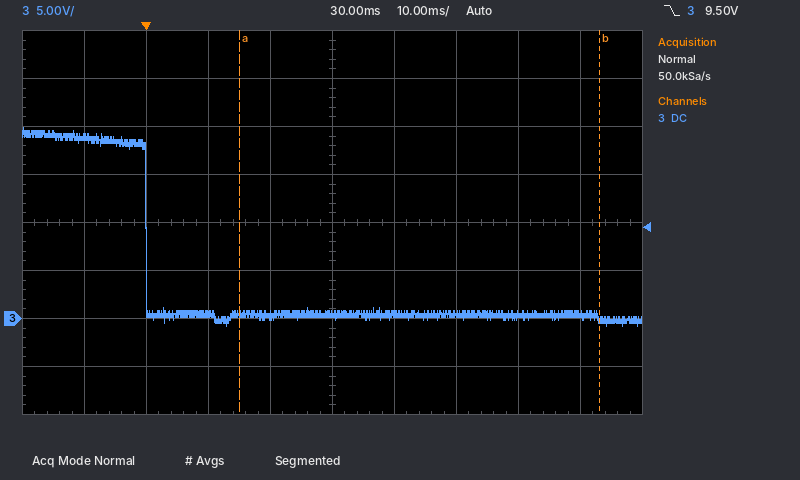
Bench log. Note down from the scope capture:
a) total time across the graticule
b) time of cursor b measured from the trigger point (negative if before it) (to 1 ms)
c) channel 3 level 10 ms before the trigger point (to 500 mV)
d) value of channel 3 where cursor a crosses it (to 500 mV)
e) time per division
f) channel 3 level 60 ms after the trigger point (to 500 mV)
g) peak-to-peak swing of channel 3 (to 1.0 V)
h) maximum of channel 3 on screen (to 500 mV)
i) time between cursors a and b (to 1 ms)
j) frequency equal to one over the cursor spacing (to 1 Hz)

100 ms
+73 ms
19.0 V
500 mV
10 ms
500 mV
21.0 V
20.0 V
58 ms
17 Hz
